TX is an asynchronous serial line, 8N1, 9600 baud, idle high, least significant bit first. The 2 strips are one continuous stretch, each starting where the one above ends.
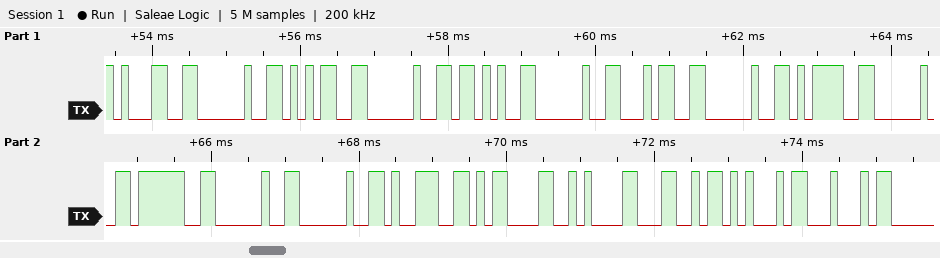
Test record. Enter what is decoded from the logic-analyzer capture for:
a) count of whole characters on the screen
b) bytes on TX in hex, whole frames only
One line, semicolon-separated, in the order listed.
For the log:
19; 0x31 0x20 0x35 0x20 0x2B 0x20 0x34 0x20 0x3D 0x20 0x3F 0x20 0x20 0x39 0x0D 0x0A 0x4C 0x45 0x44
